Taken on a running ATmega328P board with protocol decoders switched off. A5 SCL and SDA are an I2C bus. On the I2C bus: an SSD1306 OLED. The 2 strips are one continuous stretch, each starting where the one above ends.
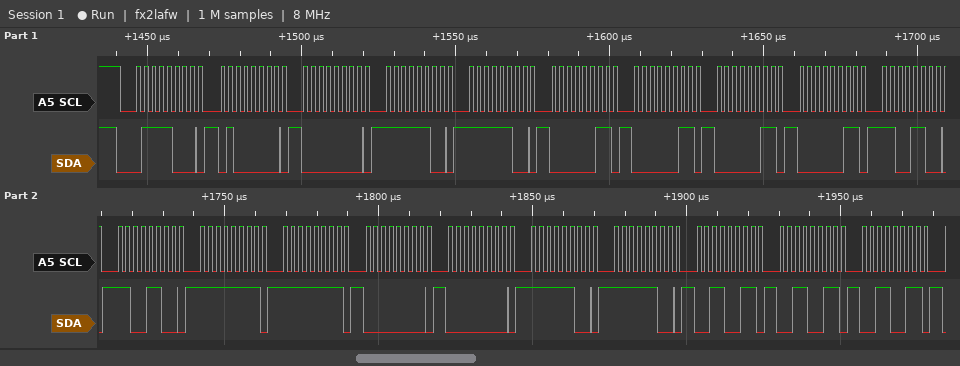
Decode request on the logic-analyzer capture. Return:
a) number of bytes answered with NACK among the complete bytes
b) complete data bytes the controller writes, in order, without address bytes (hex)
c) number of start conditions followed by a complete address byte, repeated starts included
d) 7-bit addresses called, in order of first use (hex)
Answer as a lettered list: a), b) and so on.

a) 0
b) 40 00 FC FC 03 03 03 03 CC CC FF FF 00 00 FC FC 33 33 33
c) 1
d) 0x3C
